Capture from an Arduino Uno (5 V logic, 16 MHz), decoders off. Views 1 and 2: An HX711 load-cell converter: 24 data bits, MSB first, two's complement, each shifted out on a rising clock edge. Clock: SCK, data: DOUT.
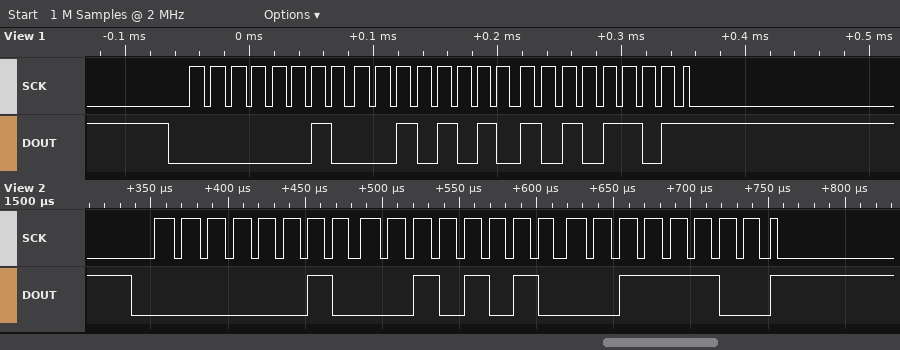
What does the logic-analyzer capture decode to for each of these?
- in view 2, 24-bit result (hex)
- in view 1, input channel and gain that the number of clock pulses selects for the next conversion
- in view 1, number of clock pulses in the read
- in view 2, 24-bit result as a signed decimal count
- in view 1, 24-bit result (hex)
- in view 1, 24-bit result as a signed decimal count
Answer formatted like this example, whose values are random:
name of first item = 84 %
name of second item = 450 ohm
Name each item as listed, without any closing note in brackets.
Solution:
in view 2, 24-bit result = 0x022A3C
in view 1, input channel and gain that the number of clock pulses selects for the next conversion = channel A, gain 128
in view 1, number of clock pulses in the read = 25
in view 2, 24-bit result as a signed decimal count = 141884
in view 1, 24-bit result = 0x022AAD
in view 1, 24-bit result as a signed decimal count = 141997
